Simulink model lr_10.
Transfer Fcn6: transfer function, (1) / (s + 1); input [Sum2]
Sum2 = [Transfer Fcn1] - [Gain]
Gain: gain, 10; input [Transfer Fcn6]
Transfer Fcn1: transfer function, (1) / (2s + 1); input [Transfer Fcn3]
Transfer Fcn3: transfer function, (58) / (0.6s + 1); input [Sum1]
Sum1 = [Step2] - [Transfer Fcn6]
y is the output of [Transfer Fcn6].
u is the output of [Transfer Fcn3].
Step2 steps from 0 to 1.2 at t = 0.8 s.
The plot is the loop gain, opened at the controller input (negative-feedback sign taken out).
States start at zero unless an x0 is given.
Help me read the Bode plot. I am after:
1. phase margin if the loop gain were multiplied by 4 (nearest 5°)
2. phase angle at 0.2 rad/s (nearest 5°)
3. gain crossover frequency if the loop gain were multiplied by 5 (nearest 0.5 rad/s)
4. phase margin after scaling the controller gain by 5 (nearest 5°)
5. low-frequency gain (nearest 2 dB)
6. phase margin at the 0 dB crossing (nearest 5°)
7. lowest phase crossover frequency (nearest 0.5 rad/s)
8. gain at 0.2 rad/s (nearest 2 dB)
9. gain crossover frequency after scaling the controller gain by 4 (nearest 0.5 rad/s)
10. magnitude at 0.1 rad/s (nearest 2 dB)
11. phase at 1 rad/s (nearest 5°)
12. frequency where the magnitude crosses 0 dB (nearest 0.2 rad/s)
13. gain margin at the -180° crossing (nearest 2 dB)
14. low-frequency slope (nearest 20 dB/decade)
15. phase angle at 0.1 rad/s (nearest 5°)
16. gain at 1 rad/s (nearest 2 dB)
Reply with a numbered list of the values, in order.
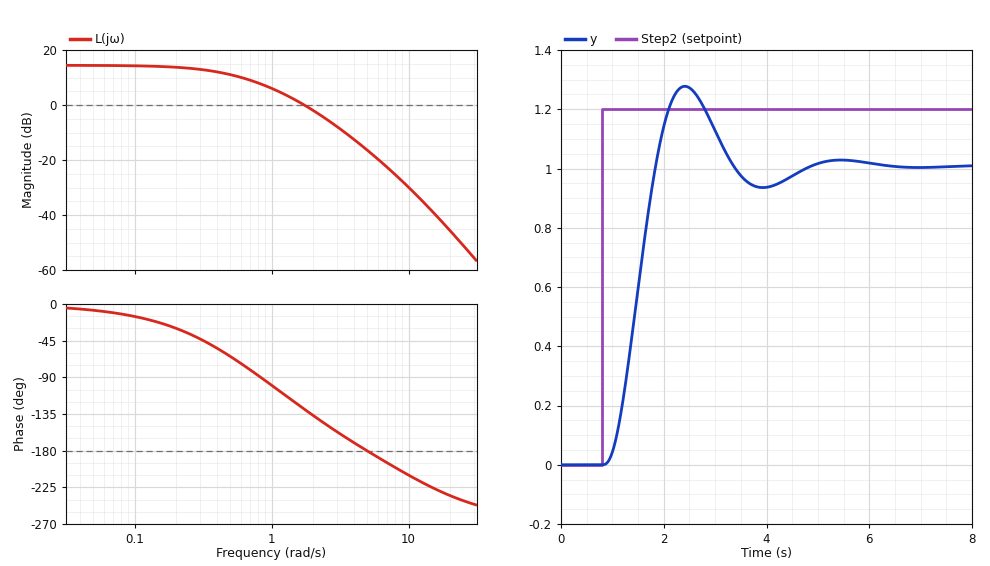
1. 10°
2. -30°
3. 4.5 rad/s
4. 5°
5. 14 dB
6. 50°
7. 5.0 rad/s
8. 14 dB
9. 4.0 rad/s
10. 14 dB
11. -100°
12. 1.8 rad/s
13. 16 dB
14. 0 dB/decade
15. -15°
16. 6 dB
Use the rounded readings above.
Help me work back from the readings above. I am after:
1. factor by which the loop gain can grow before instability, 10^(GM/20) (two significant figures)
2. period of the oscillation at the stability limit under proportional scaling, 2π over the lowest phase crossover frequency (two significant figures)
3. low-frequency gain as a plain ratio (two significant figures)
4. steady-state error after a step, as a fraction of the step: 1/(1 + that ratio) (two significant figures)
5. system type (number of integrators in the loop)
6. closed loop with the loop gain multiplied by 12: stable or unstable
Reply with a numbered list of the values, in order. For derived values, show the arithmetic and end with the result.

1. 10^(16 / 20) = 6.3
2. 2π / 5 = 1.3 s
3. 10^(14 / 20) = 5.0
4. 1 / (1 + 5) = 0.17
5. 0
6. unstable
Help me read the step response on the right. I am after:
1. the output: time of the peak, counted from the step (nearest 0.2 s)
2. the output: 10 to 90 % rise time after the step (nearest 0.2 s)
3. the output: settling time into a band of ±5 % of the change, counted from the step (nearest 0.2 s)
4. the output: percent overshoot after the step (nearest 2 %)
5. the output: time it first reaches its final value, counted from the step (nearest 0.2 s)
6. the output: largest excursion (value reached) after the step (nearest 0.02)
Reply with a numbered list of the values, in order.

1. 1.6 s
2. 0.6 s
3. 3.6 s
4. 26 %
5. 1.0 s
6. 1.28
